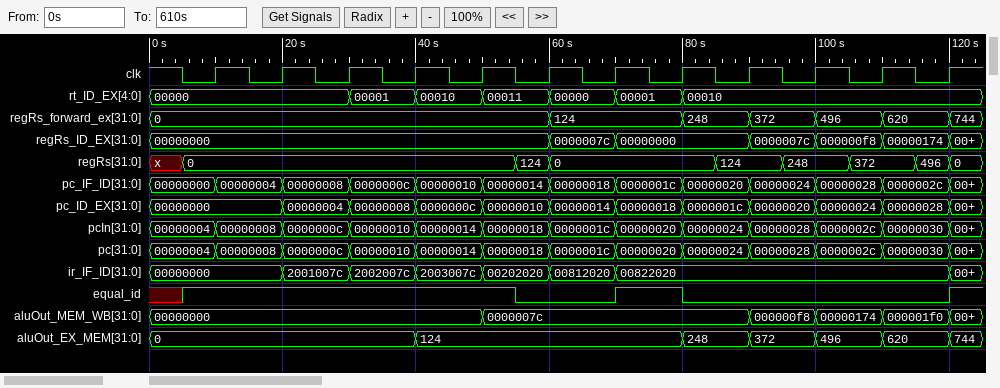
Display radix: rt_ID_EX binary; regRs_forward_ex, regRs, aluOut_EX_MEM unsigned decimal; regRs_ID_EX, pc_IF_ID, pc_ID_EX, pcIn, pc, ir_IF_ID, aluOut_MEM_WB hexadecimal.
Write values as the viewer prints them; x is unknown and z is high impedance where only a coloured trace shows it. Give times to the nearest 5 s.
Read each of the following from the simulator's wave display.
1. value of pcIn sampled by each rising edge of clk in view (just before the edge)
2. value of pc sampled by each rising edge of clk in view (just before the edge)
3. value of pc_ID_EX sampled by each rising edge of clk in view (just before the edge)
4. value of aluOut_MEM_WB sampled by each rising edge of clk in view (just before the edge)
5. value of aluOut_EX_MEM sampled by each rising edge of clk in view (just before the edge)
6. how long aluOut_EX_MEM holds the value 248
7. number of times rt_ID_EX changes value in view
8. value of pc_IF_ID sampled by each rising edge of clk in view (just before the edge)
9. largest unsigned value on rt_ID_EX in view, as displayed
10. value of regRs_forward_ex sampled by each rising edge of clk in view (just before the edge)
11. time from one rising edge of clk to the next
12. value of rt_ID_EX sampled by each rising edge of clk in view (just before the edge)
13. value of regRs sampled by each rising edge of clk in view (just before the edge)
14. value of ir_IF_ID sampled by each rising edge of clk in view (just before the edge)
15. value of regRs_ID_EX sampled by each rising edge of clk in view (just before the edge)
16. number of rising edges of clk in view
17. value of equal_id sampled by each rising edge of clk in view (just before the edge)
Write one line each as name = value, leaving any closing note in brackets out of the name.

value of pcIn sampled by each rising edge of clk in view = 00000004, 00000008, 0000000c, 00000010, 00000014, 00000018, 0000001c, 00000020, 00000024, 00000028, 0000002c, 00000030
value of pc sampled by each rising edge of clk in view = 00000004, 00000008, 0000000c, 00000010, 00000014, 00000018, 0000001c, 00000020, 00000024, 00000028, 0000002c, 00000030
value of pc_ID_EX sampled by each rising edge of clk in view = 00000000, 00000000, 00000004, 00000008, 0000000c, 00000010, 00000014, 00000018, 0000001c, 00000020, 00000024, 00000028
value of aluOut_MEM_WB sampled by each rising edge of clk in view = 00000000, 00000000, 00000000, 00000000, 00000000, 0000007c, 0000007c, 0000007c, 0000007c, 000000f8, 00000174, 000001f0
value of aluOut_EX_MEM sampled by each rising edge of clk in view = 0, 0, 0, 0, 124, 124, 124, 124, 248, 372, 496, 620
how long aluOut_EX_MEM holds the value 248 = 10 s
number of times rt_ID_EX changes value in view = 6
value of pc_IF_ID sampled by each rising edge of clk in view = 00000000, 00000004, 00000008, 0000000c, 00000010, 00000014, 00000018, 0000001c, 00000020, 00000024, 00000028, 0000002c
largest unsigned value on rt_ID_EX in view, as displayed = 00011
value of regRs_forward_ex sampled by each rising edge of clk in view = 0, 0, 0, 0, 0, 0, 124, 124, 248, 372, 496, 620
time from one rising edge of clk to the next = 10 s
value of rt_ID_EX sampled by each rising edge of clk in view = 00000, 00000, 00000, 00001, 00010, 00011, 00000, 00001, 00010, 00010, 00010, 00010
value of regRs sampled by each rising edge of clk in view = 0, 0, 0, 0, 0, 124, 0, 0, 124, 248, 372, 496
value of ir_IF_ID sampled by each rising edge of clk in view = 00000000, 00000000, 2001007c, 2002007c, 2003007c, 00202020, 00812020, 00822020, 00822020, 00822020, 00822020, 00822020
value of regRs_ID_EX sampled by each rising edge of clk in view = 00000000, 00000000, 00000000, 00000000, 00000000, 00000000, 0000007c, 00000000, 00000000, 0000007c, 000000f8, 00000174
number of rising edges of clk in view = 12
value of equal_id sampled by each rising edge of clk in view = 1 1 1 1 1 0 0 1 0 0 0 0
